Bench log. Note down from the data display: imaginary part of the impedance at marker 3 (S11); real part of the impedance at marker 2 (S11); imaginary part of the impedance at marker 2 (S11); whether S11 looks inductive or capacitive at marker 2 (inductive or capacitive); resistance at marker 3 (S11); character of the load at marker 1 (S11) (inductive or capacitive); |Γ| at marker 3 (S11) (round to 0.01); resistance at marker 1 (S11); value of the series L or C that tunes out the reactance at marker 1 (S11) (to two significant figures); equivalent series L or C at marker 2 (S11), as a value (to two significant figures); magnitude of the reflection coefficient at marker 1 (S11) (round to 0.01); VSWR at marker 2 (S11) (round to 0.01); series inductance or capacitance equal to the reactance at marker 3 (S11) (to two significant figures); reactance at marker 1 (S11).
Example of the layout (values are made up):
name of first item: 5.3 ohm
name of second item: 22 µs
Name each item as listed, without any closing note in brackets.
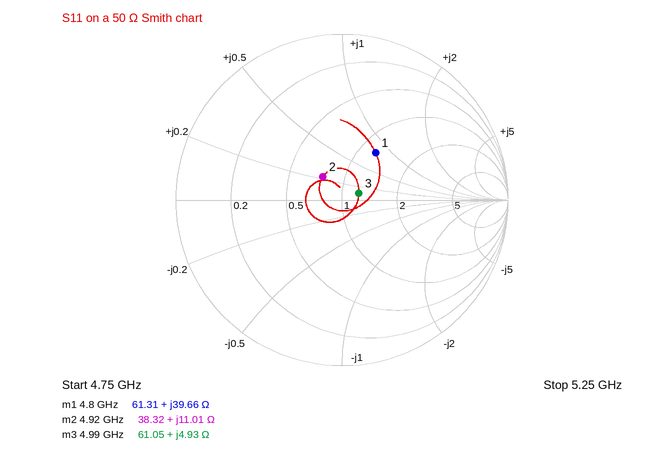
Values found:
imaginary part of the impedance at marker 3: +4.93 Ω
real part of the impedance at marker 2: 38.32 Ω
imaginary part of the impedance at marker 2: +11.01 Ω
whether S11 looks inductive or capacitive at marker 2: inductive
resistance at marker 3: 61.05 Ω
character of the load at marker 1 (S11): inductive
|Γ| at marker 3 (S11): 0.11
resistance at marker 1: 61.31 Ω
value of the series L or C that tunes out the reactance at marker 1 (S11): 840 fF
equivalent series L or C at marker 2 (S11), as a value: 360 pH
magnitude of the reflection coefficient at marker 1 (S11): 0.35
VSWR at marker 2 (S11): 1.44
series inductance or capacitance equal to the reactance at marker 3 (S11): 160 pH
reactance at marker 1: +39.66 Ω
